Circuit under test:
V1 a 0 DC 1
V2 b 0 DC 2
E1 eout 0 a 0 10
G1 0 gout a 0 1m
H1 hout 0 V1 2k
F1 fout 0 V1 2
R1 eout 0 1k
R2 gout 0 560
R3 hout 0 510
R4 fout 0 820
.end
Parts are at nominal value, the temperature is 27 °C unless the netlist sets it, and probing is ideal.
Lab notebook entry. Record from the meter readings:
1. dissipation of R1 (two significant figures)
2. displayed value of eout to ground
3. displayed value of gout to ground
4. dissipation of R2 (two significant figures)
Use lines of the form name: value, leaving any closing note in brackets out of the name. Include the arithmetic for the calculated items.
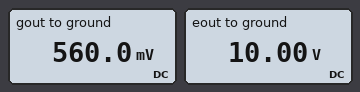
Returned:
dissipation of R1: (10 V)^2 / 1 kΩ = 100 mW
displayed value of eout to ground: 10.00 V
displayed value of gout to ground: 560.0 mV
dissipation of R2: (560 mV)^2 / 560 Ω = 560 µW
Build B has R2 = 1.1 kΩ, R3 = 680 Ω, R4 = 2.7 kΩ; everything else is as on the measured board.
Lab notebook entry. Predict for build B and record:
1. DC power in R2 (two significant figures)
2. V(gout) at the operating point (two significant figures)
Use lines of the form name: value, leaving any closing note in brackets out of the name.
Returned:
DC power in R2: 1.1 mW
V(gout) at the operating point: 1.1 V
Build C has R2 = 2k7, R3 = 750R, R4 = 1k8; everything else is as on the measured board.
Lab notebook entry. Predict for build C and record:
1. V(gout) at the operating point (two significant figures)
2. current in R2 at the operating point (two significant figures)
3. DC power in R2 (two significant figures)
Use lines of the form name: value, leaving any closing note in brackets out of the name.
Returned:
V(gout) at the operating point: 2.7 V
current in R2 at the operating point: 1.0 mA
DC power in R2: 2.7 mW
